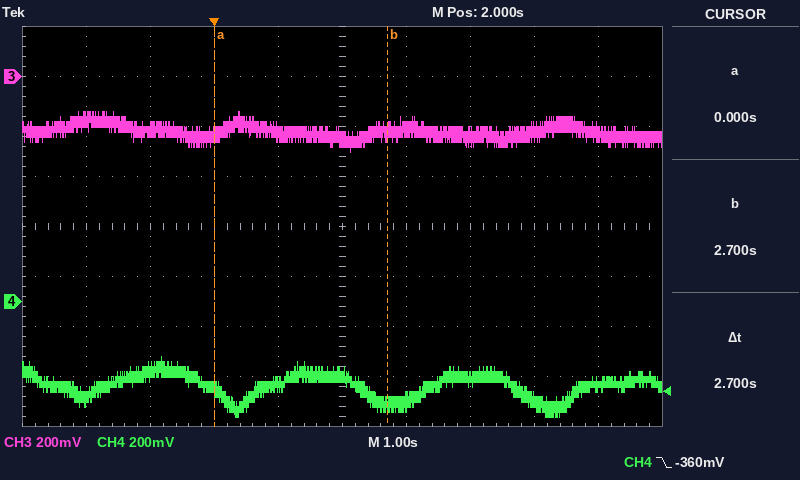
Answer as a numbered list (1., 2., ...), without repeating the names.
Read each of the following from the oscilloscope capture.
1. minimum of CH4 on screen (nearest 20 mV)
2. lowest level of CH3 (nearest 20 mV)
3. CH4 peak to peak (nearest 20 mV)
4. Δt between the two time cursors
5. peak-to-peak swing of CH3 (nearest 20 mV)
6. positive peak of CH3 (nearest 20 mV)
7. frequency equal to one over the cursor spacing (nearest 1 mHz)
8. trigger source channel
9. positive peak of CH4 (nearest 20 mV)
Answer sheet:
1. -460 mV
2. -300 mV
3. 240 mV
4. 2.7 s
5. 160 mV
6. -140 mV
7. 370 mHz
8. CH4
9. -220 mV
